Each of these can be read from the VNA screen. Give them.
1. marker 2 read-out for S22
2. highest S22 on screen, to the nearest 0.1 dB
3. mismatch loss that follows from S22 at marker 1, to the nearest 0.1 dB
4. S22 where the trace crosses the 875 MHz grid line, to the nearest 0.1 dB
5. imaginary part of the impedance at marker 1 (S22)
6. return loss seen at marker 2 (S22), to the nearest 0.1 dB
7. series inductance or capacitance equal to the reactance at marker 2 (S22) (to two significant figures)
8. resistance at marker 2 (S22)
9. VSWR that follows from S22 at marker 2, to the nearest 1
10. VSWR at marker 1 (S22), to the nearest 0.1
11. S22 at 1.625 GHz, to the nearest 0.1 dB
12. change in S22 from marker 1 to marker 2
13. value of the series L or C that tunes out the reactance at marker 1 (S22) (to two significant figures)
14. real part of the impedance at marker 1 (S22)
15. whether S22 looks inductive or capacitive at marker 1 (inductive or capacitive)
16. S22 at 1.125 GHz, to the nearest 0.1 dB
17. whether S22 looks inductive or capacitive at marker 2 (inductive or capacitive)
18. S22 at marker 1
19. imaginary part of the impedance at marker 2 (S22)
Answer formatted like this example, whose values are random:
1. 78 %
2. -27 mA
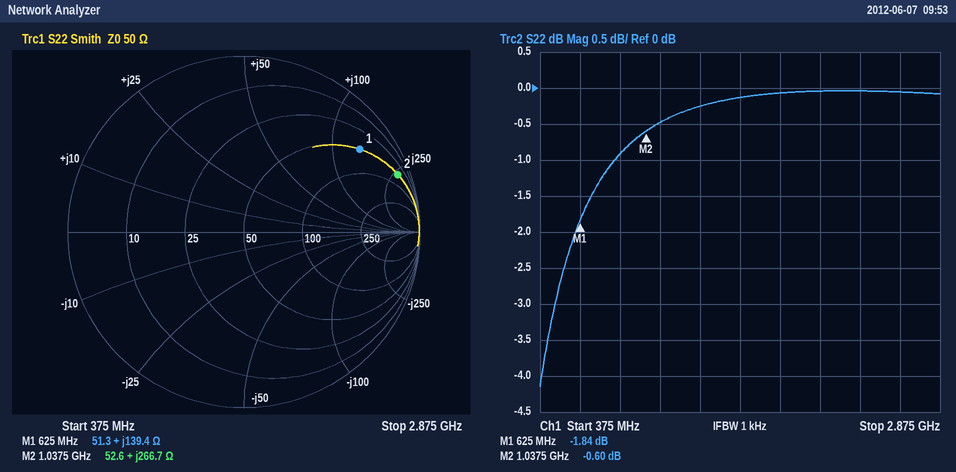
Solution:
1. -0.60 dB
2. 0.0 dB
3. 4.6 dB
4. -0.9 dB
5. +139.4 Ω
6. 0.6 dB
7. 41 nH
8. 52.6 Ω
9. 29
10. 9.5
11. -0.1 dB
12. 1.24 dB
13. 1.8 pF
14. 51.3 Ω
15. inductive
16. -0.5 dB
17. inductive
18. -1.84 dB
19. +266.7 Ω
